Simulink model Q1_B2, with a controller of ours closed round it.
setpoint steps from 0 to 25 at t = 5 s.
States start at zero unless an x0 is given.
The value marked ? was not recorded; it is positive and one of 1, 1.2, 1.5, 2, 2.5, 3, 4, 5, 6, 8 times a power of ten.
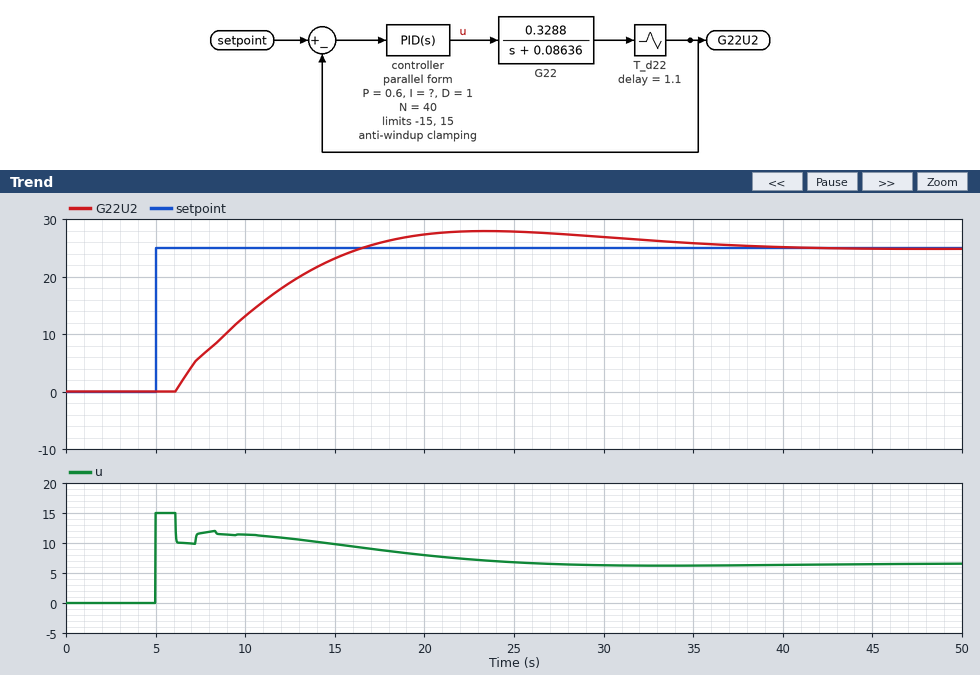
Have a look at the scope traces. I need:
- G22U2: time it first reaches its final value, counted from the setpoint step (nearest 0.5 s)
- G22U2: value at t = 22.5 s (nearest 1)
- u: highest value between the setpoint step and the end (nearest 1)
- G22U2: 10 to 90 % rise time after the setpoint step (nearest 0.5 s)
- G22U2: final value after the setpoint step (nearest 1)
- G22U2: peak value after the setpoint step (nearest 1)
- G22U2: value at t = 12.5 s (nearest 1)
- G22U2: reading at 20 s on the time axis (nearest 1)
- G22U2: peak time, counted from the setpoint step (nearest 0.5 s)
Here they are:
11.5 s
28
15
8.0 s
25
28
19
27
18.5 s
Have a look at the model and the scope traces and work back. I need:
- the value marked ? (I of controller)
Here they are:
0.1
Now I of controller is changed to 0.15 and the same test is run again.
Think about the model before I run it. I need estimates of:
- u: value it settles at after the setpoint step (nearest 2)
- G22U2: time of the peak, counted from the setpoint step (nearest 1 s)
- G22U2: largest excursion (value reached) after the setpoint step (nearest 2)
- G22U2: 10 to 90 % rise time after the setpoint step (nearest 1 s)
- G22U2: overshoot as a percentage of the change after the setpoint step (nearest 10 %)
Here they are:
6
15 s
30
6 s
20 %
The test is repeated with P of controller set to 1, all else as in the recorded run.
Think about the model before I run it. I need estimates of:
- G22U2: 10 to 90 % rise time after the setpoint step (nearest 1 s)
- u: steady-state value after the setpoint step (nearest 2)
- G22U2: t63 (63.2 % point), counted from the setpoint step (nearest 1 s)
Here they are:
8 s
6
5 s
